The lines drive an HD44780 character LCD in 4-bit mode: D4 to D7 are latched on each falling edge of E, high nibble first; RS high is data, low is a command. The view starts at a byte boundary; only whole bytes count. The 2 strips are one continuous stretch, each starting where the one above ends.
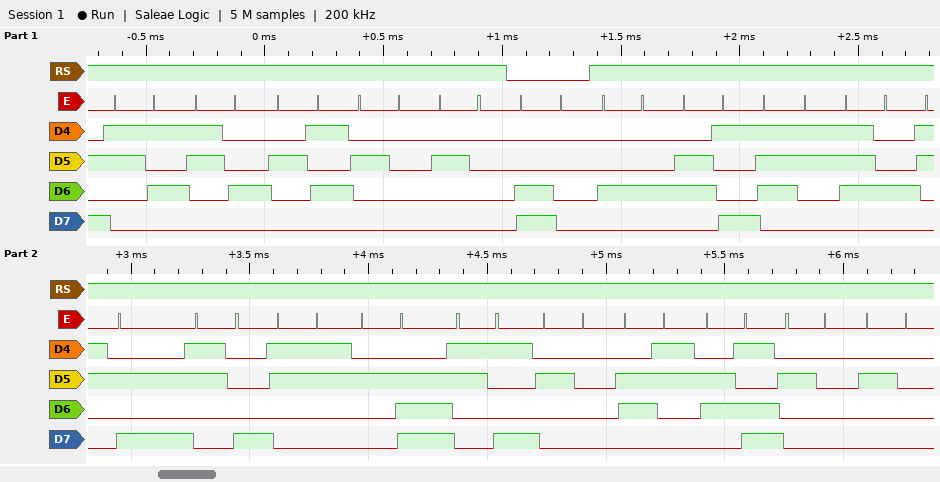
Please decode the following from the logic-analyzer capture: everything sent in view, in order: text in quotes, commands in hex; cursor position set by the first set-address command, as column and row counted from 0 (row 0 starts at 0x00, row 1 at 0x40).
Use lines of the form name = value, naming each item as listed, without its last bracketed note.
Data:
everything sent in view, in order: text in quotes, commands in hex = "54%  " 0xC0 "Dist:83.9 cm  "
cursor position set by the first set-address command, as column and row counted from 0 = column 0, row 1
